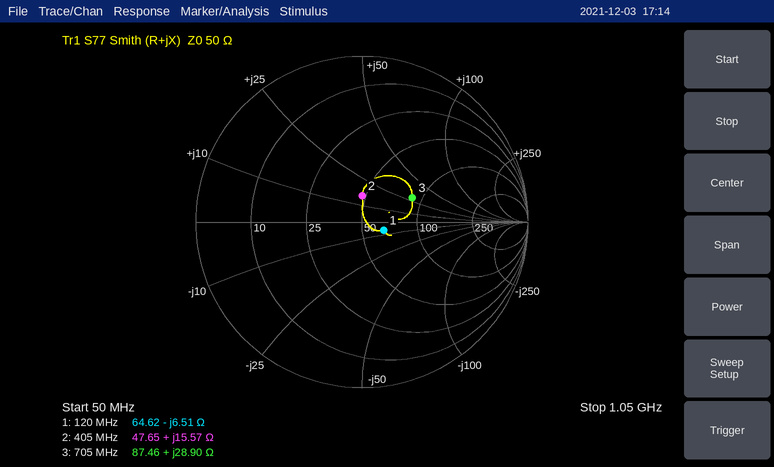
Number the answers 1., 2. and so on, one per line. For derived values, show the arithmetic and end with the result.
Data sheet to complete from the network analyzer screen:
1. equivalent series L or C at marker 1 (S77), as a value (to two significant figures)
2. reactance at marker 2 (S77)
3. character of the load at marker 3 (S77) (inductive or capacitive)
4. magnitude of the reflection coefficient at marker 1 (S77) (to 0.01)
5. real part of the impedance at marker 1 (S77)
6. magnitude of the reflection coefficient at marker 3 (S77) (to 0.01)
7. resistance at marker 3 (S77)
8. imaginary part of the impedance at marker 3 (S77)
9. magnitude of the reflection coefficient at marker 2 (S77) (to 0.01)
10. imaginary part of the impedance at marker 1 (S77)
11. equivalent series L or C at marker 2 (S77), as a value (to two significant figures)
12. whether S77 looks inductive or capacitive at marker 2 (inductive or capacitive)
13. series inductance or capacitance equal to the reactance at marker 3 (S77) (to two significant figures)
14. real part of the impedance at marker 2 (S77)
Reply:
1. C = 1/(2π × 120 MHz × 6.51 Ω) ≈ 204 pF, so 200 pF to two significant figures
2. +15.57 Ω
3. inductive
4. 0.14
5. 64.62 Ω
6. 0.34
7. 87.46 Ω
8. +28.90 Ω
9. 0.16
10. -6.51 Ω
11. L = 15.57 Ω/(2π × 405 MHz) ≈ 6.1 nH
12. inductive
13. L = 28.9 Ω/(2π × 705 MHz) ≈ 6.5 nH
14. 47.65 Ω
